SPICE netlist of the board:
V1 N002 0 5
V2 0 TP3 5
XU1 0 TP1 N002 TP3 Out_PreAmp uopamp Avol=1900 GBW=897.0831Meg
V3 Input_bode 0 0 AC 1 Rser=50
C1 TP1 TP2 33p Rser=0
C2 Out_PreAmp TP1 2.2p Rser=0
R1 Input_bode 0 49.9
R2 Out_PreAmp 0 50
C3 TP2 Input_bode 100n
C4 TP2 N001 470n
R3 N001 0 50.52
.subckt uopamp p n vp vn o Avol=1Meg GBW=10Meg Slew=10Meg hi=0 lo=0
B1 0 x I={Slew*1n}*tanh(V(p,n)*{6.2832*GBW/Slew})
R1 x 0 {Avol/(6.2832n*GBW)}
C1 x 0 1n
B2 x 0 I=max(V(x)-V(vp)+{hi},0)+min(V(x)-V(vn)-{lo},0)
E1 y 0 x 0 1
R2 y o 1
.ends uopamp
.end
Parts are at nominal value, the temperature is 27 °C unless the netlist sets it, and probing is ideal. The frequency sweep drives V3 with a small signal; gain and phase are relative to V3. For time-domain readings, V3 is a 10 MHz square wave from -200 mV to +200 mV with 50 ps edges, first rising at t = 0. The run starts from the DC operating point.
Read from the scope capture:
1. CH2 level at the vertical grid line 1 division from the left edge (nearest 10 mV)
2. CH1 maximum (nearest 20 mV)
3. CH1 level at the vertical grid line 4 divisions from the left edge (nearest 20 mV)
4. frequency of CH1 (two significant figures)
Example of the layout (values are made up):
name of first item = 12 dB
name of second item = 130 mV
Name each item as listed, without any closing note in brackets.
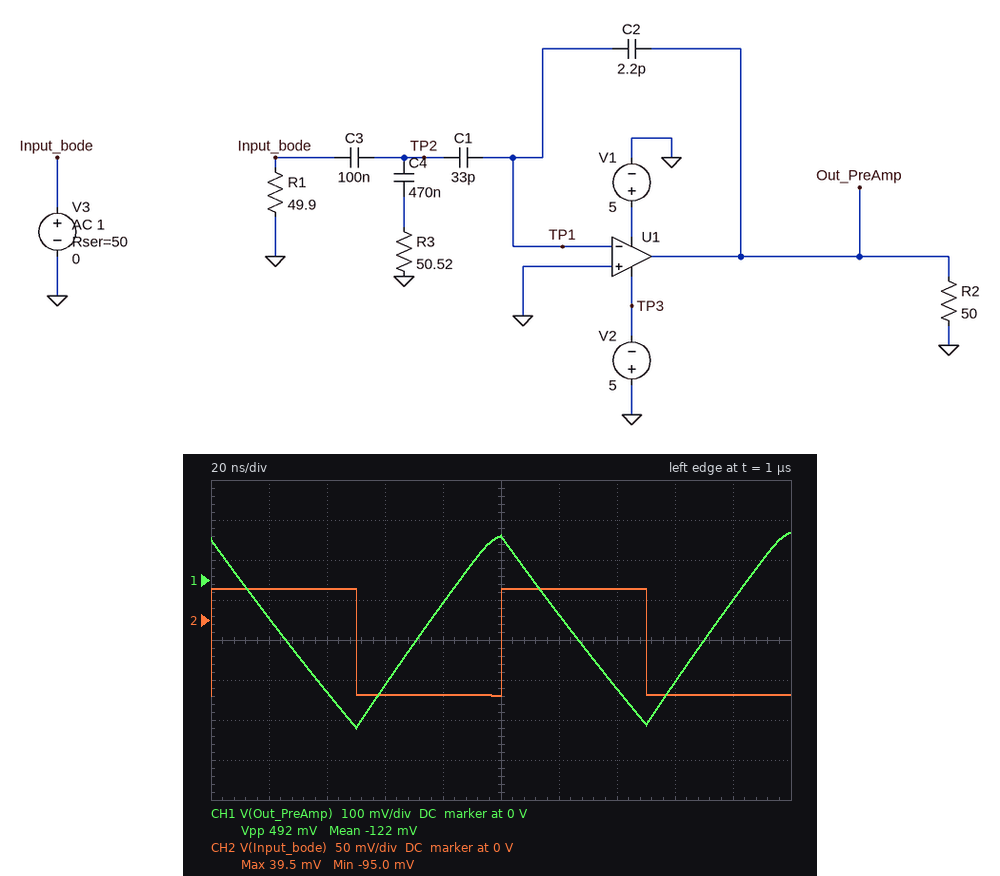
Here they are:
CH2 level at the vertical grid line 1 division from the left edge = 40 mV
CH1 maximum = 120 mV
CH1 level at the vertical grid line 4 divisions from the left edge = -60 mV
frequency of CH1 = 10 MHz
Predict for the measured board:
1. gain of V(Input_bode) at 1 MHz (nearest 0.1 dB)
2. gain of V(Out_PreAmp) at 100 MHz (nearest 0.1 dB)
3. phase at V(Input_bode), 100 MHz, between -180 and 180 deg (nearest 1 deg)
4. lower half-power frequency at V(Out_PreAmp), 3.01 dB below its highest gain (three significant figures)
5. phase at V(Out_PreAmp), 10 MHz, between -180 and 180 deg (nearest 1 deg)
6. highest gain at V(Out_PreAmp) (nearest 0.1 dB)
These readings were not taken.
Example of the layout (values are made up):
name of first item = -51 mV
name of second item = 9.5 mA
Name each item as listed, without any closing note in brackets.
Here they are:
gain of V(Input_bode) at 1 MHz = -9.5 dB
gain of V(Out_PreAmp) at 100 MHz = 6.5 dB
phase at V(Input_bode), 100 MHz, between -180 and 180 deg = -5 deg
lower half-power frequency at V(Out_PreAmp), 3.01 dB below its highest gain = 23.7 kHz
phase at V(Out_PreAmp), 10 MHz, between -180 and 180 deg = 168 deg
highest gain at V(Out_PreAmp) = 13.9 dB
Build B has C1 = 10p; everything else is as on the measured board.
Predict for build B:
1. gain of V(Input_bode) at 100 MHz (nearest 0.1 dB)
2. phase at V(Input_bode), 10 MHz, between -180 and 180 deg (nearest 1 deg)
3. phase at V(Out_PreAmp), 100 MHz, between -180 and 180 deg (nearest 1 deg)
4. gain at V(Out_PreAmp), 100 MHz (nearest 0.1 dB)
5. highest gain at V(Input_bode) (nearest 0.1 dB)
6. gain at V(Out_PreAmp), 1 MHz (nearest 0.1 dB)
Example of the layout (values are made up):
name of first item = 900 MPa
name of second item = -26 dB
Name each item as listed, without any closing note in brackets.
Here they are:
gain of V(Input_bode) at 100 MHz = -9.9 dB
phase at V(Input_bode), 10 MHz, between -180 and 180 deg = -1 deg
phase at V(Out_PreAmp), 100 MHz, between -180 and 180 deg = 143 deg
gain at V(Out_PreAmp), 100 MHz = 1.8 dB
highest gain at V(Input_bode) = -6.0 dB
gain at V(Out_PreAmp), 1 MHz = 3.6 dB
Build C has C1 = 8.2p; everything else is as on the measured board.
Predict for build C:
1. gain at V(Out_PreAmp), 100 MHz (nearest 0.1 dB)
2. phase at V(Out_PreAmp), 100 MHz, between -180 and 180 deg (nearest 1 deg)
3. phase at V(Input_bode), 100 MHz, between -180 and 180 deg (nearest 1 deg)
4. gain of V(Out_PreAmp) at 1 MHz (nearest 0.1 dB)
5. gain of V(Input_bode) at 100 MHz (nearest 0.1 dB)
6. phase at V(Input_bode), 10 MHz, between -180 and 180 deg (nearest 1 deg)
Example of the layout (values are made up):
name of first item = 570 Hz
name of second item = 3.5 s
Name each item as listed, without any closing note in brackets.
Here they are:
gain at V(Out_PreAmp), 100 MHz = 0.5 dB
phase at V(Out_PreAmp), 100 MHz, between -180 and 180 deg = 148 deg
phase at V(Input_bode), 100 MHz, between -180 and 180 deg = -4 deg
gain of V(Out_PreAmp) at 1 MHz = 1.9 dB
gain of V(Input_bode) at 100 MHz = -9.8 dB
phase at V(Input_bode), 10 MHz, between -180 and 180 deg = -1 deg
